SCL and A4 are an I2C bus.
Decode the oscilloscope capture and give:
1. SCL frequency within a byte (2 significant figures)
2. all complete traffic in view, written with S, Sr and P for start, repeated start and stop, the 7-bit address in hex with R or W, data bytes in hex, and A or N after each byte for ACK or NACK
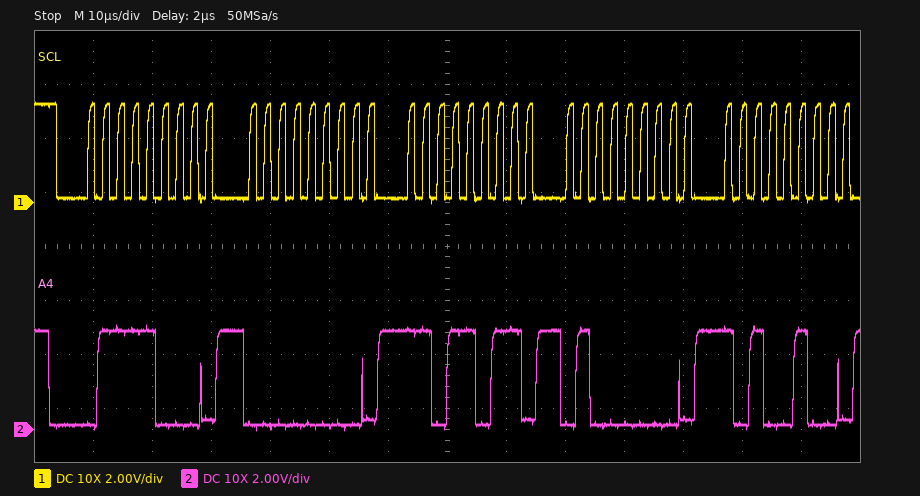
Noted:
400 kHz
S 3CW A 00 A DB A 40 A A4 A
